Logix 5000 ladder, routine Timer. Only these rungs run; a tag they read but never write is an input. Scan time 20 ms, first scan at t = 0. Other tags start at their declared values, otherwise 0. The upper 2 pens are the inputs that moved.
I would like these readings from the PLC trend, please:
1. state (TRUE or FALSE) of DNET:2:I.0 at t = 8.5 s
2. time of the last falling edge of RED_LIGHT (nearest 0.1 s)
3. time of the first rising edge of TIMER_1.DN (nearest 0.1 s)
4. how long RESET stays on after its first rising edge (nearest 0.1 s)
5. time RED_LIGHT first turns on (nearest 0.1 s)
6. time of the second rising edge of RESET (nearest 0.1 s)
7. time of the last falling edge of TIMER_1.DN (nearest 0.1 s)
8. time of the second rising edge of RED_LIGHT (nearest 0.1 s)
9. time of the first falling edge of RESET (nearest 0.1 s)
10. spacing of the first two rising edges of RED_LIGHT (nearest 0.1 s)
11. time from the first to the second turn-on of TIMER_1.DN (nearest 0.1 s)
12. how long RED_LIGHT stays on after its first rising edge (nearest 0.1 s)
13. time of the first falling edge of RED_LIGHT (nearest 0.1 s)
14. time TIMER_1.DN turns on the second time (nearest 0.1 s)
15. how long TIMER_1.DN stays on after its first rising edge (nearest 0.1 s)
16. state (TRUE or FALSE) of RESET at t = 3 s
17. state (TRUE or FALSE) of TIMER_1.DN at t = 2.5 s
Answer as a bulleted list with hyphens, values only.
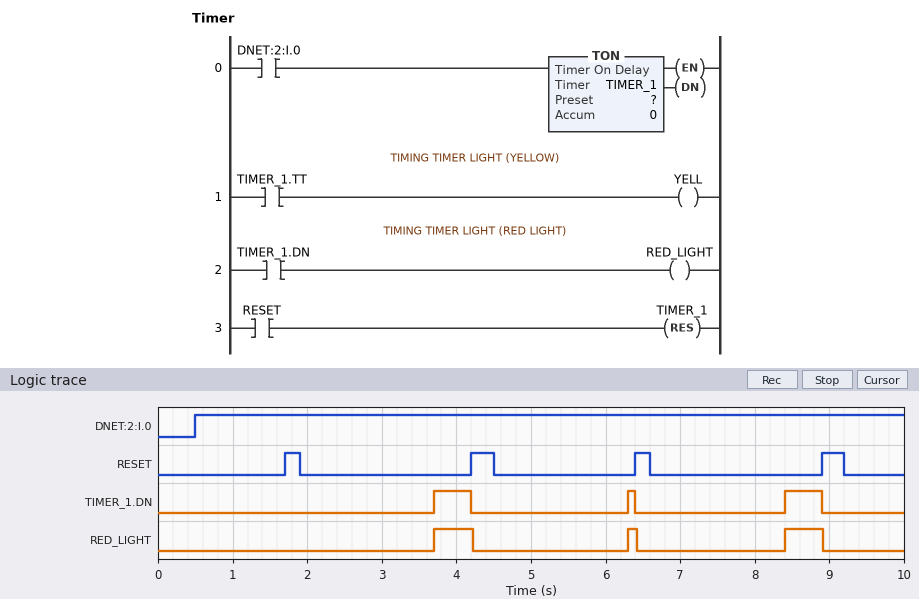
- TRUE
- 8.9 s
- 3.7 s
- 0.2 s
- 3.7 s
- 4.2 s
- 8.9 s
- 6.3 s
- 1.9 s
- 2.6 s
- 2.6 s
- 0.5 s
- 4.2 s
- 6.3 s
- 0.5 s
- FALSE
- FALSE
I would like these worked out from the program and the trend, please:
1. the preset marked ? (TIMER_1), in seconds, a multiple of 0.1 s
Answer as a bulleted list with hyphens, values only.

- 1.8 s
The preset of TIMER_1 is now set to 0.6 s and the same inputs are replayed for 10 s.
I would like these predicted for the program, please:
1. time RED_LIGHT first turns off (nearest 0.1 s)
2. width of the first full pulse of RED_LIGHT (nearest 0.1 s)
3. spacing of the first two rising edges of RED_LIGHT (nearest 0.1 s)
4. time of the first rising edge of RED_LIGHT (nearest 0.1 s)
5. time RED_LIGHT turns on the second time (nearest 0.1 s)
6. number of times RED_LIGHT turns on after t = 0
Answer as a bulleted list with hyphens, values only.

- 1.7 s
- 0.6 s
- 1.4 s
- 1.1 s
- 2.5 s
- 5
